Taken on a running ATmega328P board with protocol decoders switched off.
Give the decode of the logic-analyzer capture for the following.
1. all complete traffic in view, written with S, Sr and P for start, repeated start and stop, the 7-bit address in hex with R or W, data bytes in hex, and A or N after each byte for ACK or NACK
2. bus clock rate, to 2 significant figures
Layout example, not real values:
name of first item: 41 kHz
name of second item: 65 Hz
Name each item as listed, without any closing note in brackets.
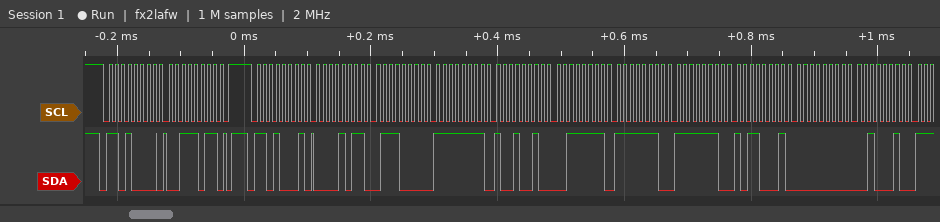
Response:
all complete traffic in view, written with S, Sr and P for start, repeated start and stop, the 7-bit address in hex with R or W, data bytes in hex, and A or N after each byte for ACK or NACK: S 68W A 3B A P S 68R A 0B A 70 A FF A 92 A 3F A FE A FE A B1 A 00 A 22 A
bus clock rate, to 2 significant figures: 100 kHz
